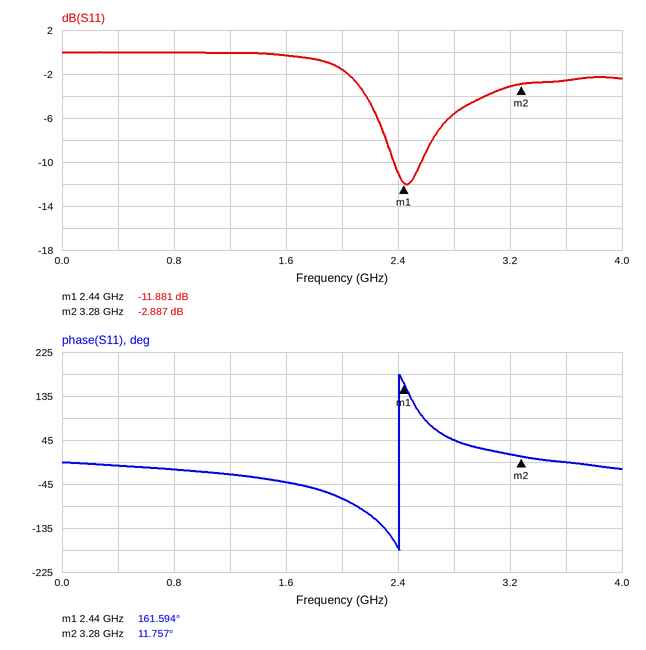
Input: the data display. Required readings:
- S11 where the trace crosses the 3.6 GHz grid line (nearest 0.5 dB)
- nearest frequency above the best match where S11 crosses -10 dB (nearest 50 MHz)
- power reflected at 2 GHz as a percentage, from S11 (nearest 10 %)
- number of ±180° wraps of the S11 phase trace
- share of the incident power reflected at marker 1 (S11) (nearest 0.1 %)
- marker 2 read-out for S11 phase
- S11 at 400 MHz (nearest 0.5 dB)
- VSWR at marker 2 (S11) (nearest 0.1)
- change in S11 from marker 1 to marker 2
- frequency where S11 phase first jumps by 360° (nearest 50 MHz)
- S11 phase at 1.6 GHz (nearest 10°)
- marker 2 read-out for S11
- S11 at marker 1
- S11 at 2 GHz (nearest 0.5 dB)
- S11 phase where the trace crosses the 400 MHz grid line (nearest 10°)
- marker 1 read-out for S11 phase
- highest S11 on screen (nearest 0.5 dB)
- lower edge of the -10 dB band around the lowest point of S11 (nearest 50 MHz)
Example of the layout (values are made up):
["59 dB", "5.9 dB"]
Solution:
["-2.5 dB", "2.55 GHz", "70 %", "1", "6.5 %", "11.757°", "0.0 dB", "6.1", "8.994 dB", "2.40 GHz", "-40°", "-2.887 dB", "-11.881 dB", "-1.5 dB", "-10°", "161.594°", "0.0 dB", "2.35 GHz"]
